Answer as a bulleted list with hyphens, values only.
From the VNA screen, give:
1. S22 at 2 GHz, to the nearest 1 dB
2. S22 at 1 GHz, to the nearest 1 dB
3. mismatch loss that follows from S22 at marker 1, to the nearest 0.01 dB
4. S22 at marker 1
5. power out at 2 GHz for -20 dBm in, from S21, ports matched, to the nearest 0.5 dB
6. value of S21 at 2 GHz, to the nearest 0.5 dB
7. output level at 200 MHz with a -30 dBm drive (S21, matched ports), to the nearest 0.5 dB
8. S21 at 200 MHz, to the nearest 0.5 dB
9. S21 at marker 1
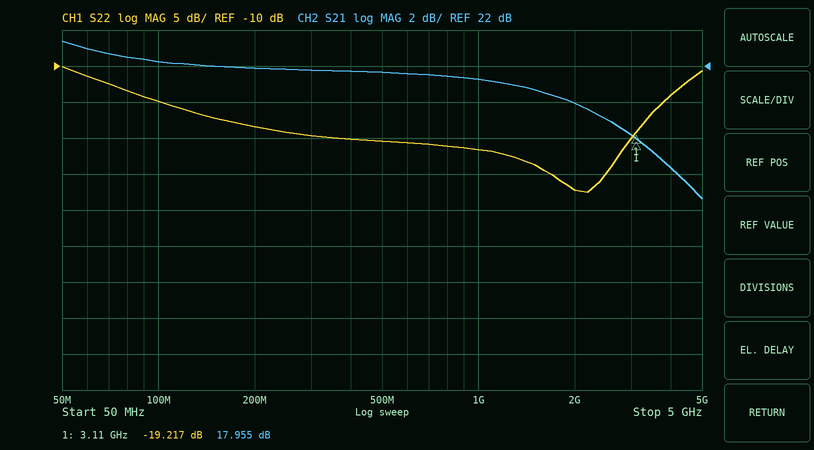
- -27 dB
- -22 dB
- 0.05 dB
- -19.217 dB
- 0.0 dBm
- 20.0 dB
- -8.0 dBm
- 22.0 dB
- 17.955 dB
